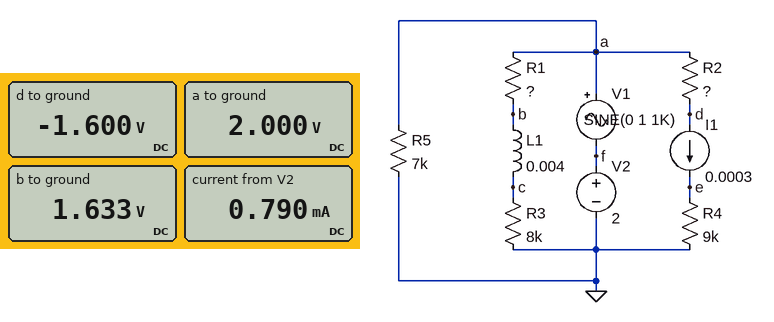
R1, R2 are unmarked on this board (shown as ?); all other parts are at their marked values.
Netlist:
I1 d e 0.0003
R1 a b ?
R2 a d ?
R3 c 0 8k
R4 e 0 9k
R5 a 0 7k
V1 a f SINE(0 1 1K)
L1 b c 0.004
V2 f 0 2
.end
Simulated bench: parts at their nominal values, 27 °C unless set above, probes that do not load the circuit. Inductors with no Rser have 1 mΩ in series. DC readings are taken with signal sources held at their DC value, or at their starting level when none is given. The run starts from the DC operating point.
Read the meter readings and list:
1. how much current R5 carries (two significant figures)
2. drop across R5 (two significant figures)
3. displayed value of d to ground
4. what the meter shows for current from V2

290 µA
2.0 V
-1.600 V
0.790 mA
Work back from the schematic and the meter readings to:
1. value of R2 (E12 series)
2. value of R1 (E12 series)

12 kΩ
1.8 kΩ
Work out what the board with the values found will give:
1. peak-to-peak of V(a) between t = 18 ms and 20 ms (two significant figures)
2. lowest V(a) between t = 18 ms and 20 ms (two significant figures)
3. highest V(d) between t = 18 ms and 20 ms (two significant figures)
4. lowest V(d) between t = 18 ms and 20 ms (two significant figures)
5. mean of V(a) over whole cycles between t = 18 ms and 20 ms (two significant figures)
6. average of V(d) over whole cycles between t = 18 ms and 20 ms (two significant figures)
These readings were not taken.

2.0 V
1.0 V
-600 mV
-2.6 V
2.0 V
-1.6 V
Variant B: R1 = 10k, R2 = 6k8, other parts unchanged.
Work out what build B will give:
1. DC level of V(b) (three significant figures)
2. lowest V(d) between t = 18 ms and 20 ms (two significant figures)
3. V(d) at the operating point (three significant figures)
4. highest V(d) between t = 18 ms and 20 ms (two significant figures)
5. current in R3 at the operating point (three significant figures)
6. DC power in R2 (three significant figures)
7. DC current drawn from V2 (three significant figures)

889 mV
-1.0 V
-40.0 mV
960 mV
111 µA
612 µW
697 µA
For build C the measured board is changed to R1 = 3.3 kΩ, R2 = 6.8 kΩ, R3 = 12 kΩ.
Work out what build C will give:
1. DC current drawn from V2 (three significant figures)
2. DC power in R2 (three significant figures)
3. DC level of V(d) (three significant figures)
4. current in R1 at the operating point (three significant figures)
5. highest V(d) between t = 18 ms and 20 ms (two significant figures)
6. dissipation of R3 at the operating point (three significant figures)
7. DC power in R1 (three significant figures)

716 µA
612 µW
-40.0 mV
131 µA
960 mV
205 µW
56.4 µW
